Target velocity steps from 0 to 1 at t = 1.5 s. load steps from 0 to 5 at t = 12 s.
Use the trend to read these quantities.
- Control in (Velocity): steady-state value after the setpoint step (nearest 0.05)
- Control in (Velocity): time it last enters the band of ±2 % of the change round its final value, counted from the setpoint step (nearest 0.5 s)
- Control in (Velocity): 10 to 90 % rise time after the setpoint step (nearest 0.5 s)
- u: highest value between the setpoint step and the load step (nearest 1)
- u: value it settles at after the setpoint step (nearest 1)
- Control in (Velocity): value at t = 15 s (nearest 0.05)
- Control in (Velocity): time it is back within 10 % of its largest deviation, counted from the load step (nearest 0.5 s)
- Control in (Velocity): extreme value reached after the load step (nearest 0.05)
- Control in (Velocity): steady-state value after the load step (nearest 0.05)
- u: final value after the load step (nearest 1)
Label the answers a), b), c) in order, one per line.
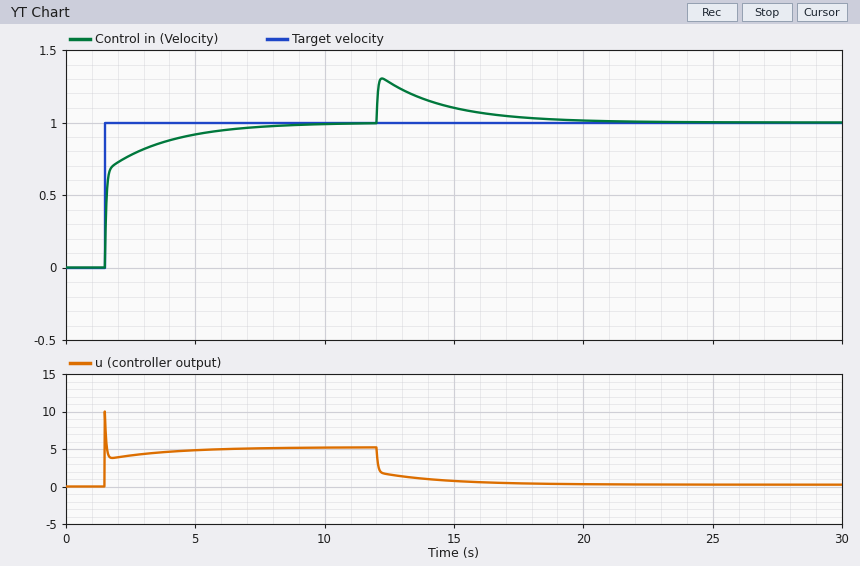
a) 1.00
b) 7.0 s
c) 3.0 s
d) 10
e) 5
f) 1.10
g) 6.0 s
h) 1.30
i) 1.00
j) 0
